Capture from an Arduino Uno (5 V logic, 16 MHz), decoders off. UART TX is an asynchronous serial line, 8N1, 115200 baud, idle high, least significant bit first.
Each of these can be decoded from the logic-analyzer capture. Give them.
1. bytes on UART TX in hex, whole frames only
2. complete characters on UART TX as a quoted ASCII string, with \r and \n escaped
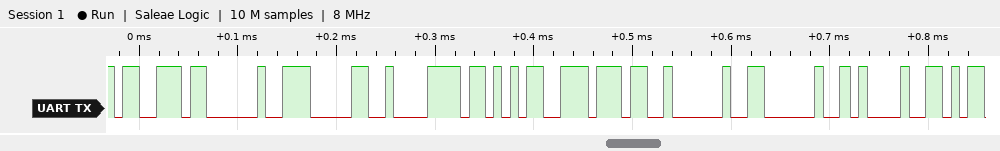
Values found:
0x73 0x20 0x30 0x78 0x35 0x37 0x20 0x20 0x21
"s 0x57  !"
